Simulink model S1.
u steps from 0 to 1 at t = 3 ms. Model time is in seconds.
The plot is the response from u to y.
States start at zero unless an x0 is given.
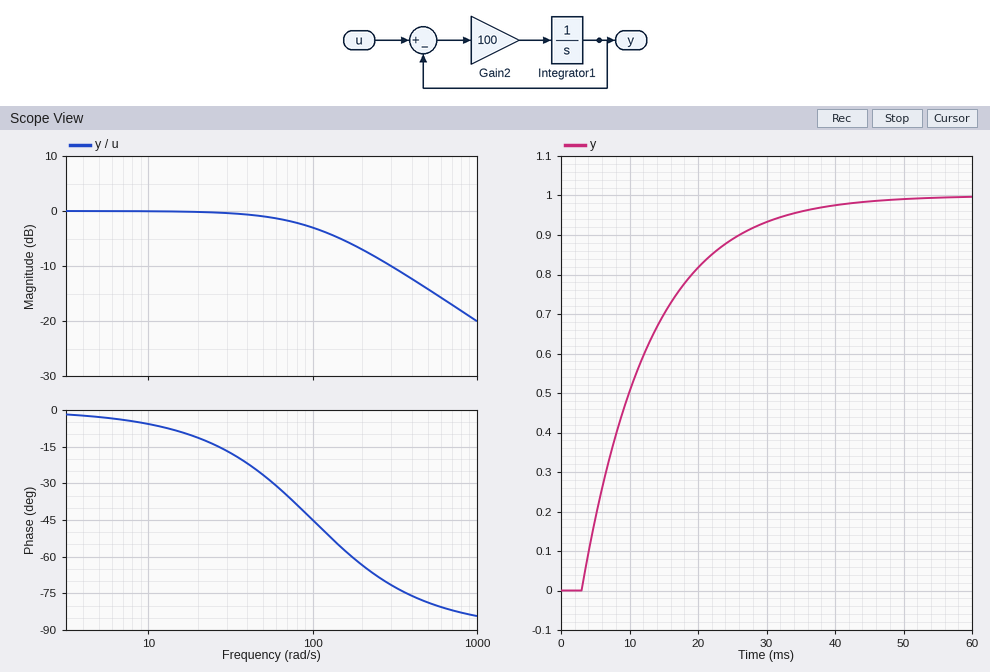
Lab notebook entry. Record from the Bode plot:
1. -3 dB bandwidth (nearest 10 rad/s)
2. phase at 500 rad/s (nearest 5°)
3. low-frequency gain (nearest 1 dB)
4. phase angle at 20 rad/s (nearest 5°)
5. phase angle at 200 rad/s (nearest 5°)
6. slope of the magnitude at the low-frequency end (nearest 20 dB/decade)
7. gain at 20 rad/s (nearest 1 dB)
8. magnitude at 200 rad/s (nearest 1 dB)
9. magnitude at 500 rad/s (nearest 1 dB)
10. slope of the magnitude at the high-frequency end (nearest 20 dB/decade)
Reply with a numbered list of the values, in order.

1. 100 rad/s
2. -80°
3. 0 dB
4. -10°
5. -65°
6. 0 dB/decade
7. 0 dB
8. -7 dB
9. -14 dB
10. -20 dB/decade
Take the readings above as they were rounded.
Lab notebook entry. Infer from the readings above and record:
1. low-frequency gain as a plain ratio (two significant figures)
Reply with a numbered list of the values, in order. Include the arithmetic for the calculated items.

1. 10^(0 / 20) = 1.0
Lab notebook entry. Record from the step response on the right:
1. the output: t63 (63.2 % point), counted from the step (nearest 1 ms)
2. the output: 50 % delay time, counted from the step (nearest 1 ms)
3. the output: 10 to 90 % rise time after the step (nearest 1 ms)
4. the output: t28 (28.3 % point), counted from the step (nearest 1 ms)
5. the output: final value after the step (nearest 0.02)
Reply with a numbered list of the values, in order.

1. 10 ms
2. 7 ms
3. 22 ms
4. 3 ms
5. 1.00
